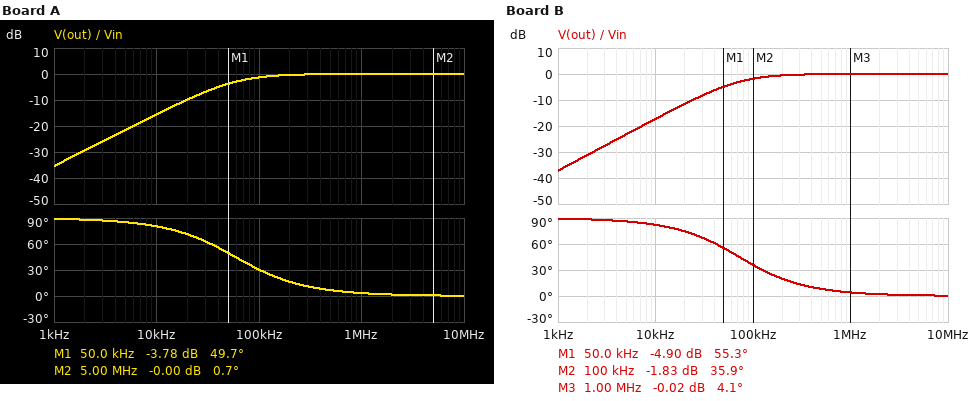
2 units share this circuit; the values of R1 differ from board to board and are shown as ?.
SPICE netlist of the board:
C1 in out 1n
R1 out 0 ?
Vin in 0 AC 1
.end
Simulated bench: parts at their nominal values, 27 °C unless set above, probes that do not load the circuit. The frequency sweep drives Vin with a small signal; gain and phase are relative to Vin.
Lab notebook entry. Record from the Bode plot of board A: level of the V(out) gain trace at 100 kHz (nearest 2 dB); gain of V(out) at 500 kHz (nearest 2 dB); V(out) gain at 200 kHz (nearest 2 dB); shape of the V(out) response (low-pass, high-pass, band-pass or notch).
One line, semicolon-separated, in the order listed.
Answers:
-2 dB; 0 dB; 0 dB; high-pass
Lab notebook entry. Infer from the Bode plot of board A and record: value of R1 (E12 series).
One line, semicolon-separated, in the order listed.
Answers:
2.7 kΩ
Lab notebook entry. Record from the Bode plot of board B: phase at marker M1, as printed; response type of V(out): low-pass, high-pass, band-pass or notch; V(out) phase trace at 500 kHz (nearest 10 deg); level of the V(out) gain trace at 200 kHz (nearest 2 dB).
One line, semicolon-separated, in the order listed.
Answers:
55.3 deg; high-pass; 10 deg; 0 dB
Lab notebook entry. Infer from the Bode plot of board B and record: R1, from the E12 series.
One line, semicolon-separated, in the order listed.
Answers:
2.2 kΩ
